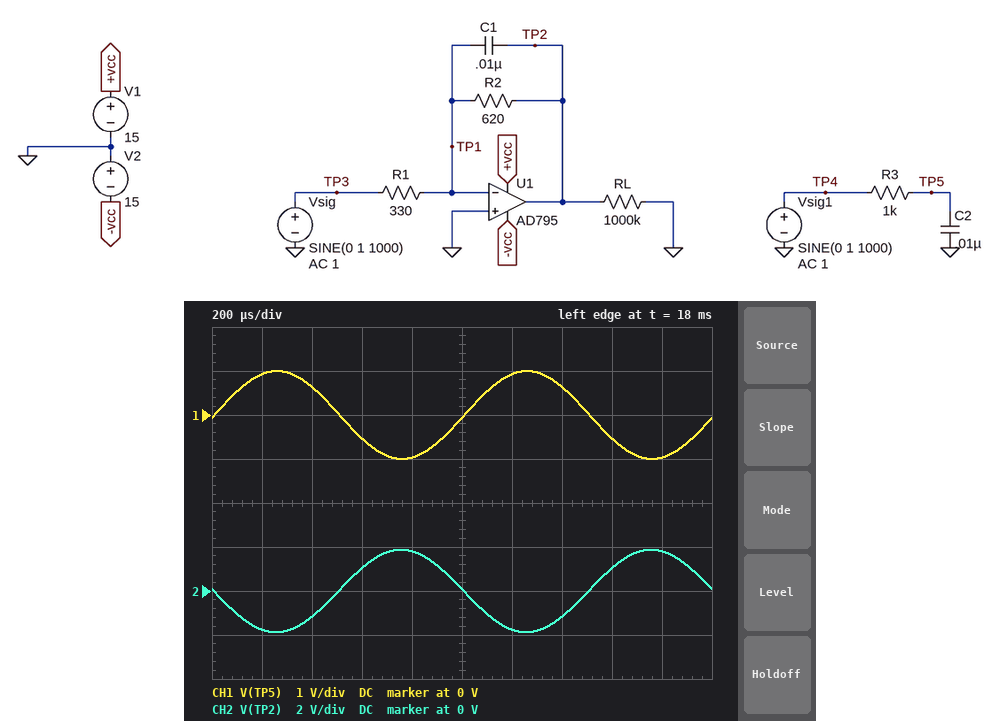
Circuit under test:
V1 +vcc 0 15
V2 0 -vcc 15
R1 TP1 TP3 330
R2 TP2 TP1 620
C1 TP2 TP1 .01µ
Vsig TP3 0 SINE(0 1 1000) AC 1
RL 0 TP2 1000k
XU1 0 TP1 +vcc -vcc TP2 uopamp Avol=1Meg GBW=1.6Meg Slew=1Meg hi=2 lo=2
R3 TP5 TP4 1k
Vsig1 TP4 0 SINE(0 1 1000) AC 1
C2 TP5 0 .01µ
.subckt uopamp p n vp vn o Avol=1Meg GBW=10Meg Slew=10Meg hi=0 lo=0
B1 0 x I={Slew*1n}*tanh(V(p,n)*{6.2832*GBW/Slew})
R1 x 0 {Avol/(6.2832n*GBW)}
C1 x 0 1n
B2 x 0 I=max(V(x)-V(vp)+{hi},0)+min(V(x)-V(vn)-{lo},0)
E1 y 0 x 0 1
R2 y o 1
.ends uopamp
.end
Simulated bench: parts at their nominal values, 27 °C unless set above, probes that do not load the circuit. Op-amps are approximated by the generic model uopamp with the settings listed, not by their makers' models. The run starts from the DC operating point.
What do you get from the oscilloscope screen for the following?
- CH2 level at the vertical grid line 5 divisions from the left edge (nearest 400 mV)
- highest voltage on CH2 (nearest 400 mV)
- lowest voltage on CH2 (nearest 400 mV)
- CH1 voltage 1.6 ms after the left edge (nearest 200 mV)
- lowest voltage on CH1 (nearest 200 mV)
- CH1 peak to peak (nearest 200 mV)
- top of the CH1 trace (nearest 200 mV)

0 V
2.0 V
-2.0 V
-600 mV
-1.0 V
2.0 V
1.0 V
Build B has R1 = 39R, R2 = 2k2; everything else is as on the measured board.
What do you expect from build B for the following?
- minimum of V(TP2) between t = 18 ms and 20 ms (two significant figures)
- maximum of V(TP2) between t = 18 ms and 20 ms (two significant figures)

-13 V
13 V
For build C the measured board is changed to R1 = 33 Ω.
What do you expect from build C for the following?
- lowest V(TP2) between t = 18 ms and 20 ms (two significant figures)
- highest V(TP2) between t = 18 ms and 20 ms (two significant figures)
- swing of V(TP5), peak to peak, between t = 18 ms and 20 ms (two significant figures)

-13 V
13 V
2.0 V
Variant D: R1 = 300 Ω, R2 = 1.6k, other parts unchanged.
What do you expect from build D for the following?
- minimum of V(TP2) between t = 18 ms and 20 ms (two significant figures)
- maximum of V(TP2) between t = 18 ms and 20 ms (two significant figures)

-5.3 V
5.3 V
